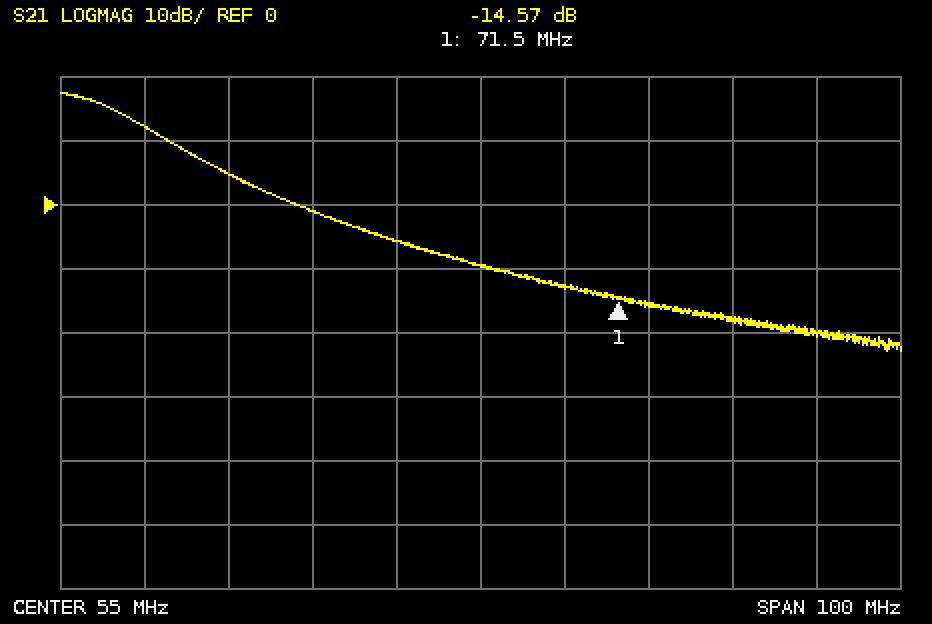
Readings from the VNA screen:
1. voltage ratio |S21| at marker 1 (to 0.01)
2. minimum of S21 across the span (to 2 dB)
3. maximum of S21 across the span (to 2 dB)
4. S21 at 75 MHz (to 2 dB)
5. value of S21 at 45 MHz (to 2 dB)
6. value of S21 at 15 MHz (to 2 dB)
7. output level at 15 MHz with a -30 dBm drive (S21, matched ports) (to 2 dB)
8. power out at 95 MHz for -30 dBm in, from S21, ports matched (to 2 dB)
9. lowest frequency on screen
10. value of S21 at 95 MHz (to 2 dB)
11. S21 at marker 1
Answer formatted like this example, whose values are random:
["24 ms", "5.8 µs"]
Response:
["0.19", "-22 dB", "18 dB", "-16 dB", "-6 dB", "12 dB", "-18 dBm", "-50 dBm", "5 MHz", "-20 dB", "-14.57 dB"]
